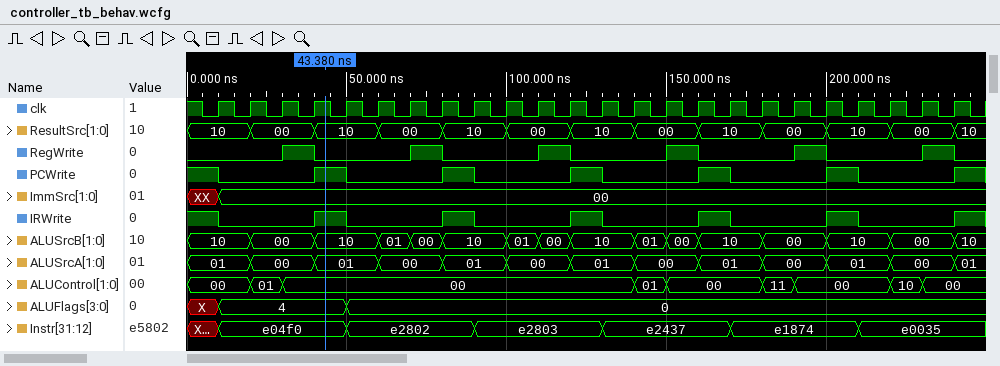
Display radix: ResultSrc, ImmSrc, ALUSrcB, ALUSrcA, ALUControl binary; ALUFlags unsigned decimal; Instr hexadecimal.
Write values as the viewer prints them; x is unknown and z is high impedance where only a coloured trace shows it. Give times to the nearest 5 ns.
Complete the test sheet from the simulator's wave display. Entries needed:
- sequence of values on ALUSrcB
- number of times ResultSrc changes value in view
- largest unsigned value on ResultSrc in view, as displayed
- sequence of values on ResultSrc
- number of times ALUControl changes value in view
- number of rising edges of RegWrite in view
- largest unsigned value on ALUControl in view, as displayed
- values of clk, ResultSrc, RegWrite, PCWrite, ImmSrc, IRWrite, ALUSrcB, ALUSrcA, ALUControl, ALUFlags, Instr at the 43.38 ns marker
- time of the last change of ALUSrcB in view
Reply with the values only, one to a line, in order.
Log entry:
10, 00, 10, 01, 00, 10, 01, 00, 10, 01, 00, 10, 00, 10, 00, 10
12
10
10, 00, 10, 00, 10, 00, 10, 00, 10, 00, 10, 00, 10
8
6
11
clk=1, ResultSrc=10, RegWrite=0, PCWrite=1, ImmSrc=00, IRWrite=1, ALUSrcB=10, ALUSrcA=01, ALUControl=00, ALUFlags=4, Instr=e04f0
240 ns
